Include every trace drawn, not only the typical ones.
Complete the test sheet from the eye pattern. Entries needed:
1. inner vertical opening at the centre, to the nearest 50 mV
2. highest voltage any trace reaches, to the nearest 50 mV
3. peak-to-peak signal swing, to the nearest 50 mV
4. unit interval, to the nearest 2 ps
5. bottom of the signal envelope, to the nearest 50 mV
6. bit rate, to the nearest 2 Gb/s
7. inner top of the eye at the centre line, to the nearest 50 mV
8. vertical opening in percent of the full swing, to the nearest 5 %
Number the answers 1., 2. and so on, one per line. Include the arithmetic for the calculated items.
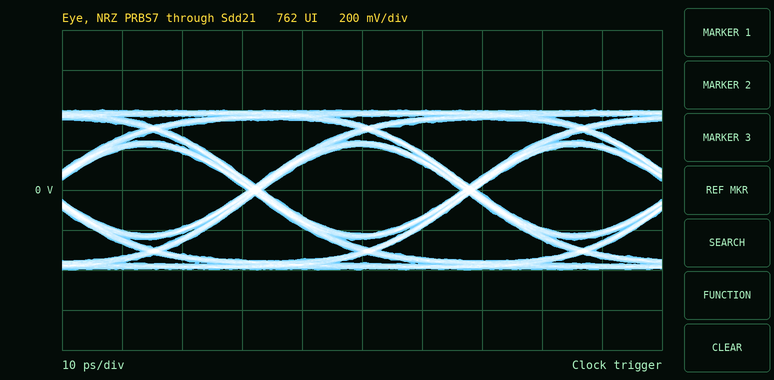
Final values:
1. 450 mV
2. 400 mV
3. 800 mV
4. 36 ps
5. -400 mV
6. 28 Gb/s
7. 200 mV
8. 450 mV / 800 mV ≈ 56.2 %, so 55 % to the nearest 5 %
